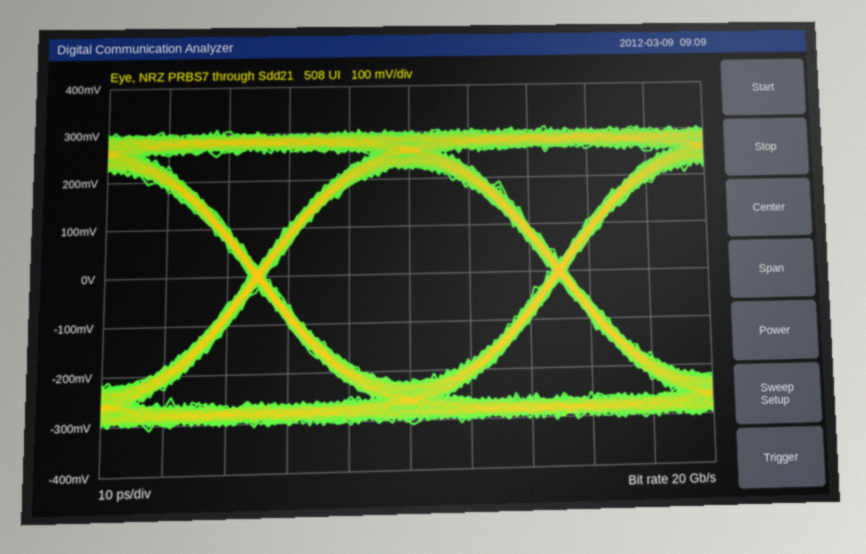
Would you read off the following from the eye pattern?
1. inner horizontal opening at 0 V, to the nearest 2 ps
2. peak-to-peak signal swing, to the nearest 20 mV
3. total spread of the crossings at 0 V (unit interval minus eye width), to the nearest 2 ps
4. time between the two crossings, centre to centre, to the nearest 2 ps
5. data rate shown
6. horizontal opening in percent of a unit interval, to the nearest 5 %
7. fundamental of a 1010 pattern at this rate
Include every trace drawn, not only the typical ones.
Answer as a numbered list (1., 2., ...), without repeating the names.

1. 48 ps
2. 620 mV
3. 2 ps
4. 50 ps
5. 20 Gb/s
6. 95 %
7. 10 GHz
